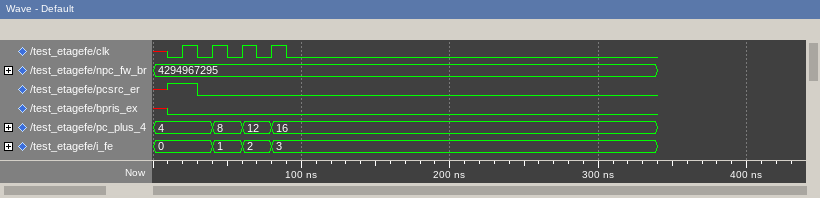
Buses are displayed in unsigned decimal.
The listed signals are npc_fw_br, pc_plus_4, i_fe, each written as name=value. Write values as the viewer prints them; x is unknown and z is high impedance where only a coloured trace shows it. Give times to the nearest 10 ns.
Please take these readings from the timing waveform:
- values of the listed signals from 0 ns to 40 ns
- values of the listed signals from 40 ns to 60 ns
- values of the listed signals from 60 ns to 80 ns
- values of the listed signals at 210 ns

npc_fw_br=4294967295, pc_plus_4=4, i_fe=0
npc_fw_br=4294967295, pc_plus_4=8, i_fe=1
npc_fw_br=4294967295, pc_plus_4=12, i_fe=2
npc_fw_br=4294967295, pc_plus_4=16, i_fe=3
